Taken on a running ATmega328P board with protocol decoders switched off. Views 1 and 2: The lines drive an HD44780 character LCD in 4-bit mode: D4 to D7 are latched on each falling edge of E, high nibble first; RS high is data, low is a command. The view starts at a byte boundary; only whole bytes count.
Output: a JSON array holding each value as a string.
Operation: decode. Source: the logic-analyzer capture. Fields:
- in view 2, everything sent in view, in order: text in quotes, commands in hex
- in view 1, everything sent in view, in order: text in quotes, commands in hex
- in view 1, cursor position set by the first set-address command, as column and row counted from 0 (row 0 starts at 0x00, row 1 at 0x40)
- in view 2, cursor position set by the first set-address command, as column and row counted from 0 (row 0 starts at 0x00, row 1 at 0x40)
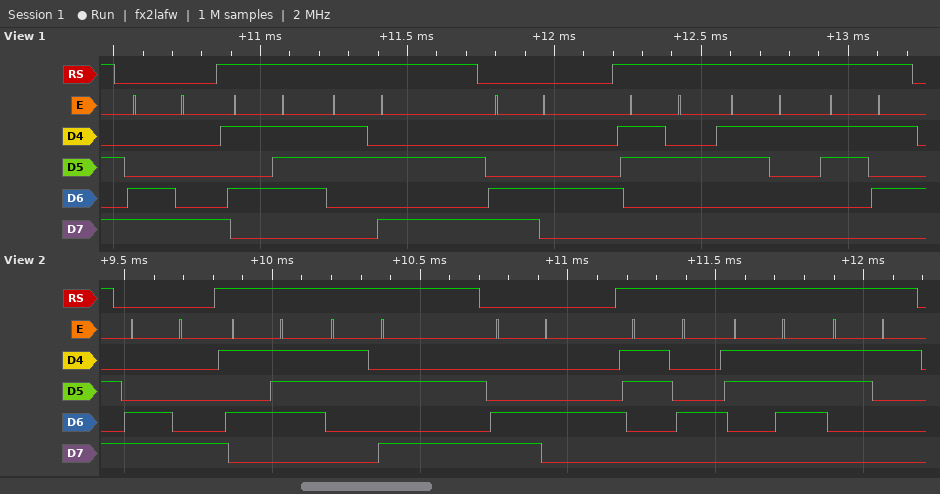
["0xC8 \"W:\" 0xC4 \"471\"", "0xC8 \"W:\" 0xC4 \"215\"", "column 8, row 1", "column 8, row 1"]
